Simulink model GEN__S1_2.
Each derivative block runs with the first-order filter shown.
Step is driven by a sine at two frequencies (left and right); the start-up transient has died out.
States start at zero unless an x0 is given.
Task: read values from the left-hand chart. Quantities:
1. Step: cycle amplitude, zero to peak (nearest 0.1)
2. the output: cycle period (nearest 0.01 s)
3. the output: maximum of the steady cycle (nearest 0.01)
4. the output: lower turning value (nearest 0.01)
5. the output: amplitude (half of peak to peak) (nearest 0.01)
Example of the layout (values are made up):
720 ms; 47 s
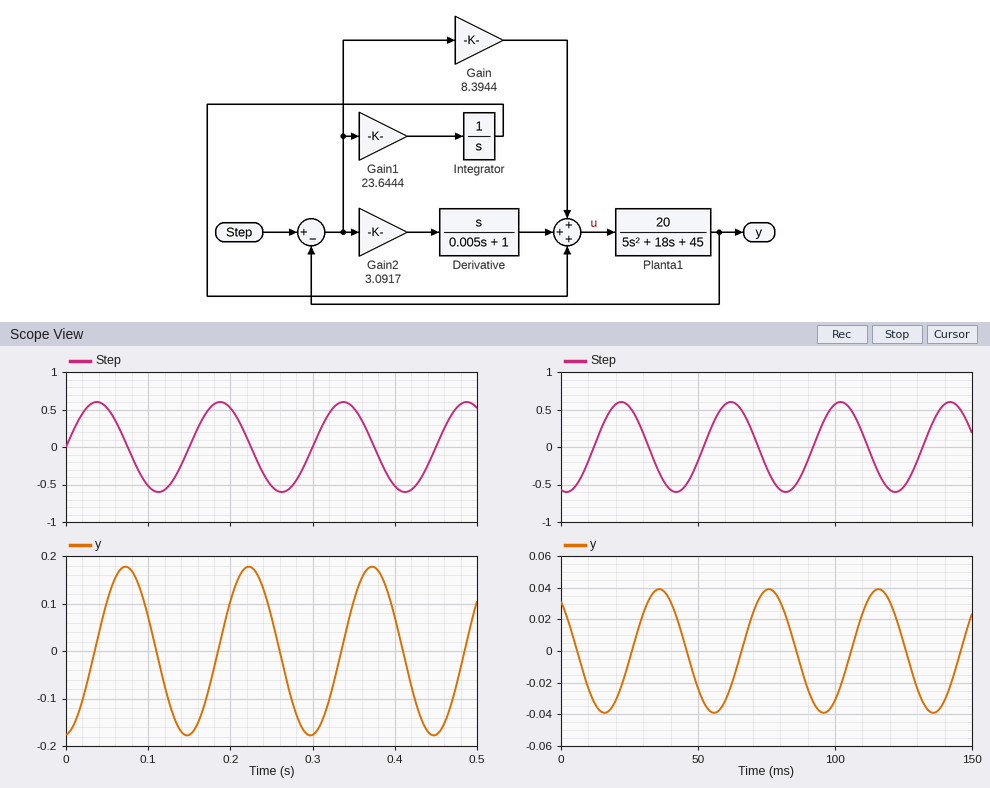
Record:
0.6; 0.15 s; 0.18; -0.18; 0.18
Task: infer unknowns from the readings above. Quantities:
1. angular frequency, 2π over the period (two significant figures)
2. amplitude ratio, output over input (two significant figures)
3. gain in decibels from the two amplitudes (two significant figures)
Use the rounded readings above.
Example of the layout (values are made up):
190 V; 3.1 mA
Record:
42 rad/s; 0.30; -10 dB
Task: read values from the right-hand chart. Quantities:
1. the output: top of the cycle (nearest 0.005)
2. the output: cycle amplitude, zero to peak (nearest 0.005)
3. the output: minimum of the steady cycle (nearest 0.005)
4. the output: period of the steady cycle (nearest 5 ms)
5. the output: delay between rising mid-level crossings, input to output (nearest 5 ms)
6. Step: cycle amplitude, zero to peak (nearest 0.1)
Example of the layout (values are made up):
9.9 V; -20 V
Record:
0.040; 0.040; -0.040; 40 ms; 15 ms; 0.6
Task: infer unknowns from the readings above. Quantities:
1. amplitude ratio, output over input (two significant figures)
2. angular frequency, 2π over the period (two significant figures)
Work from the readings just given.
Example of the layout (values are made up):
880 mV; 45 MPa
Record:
0.067; 0.16 rad/ms
